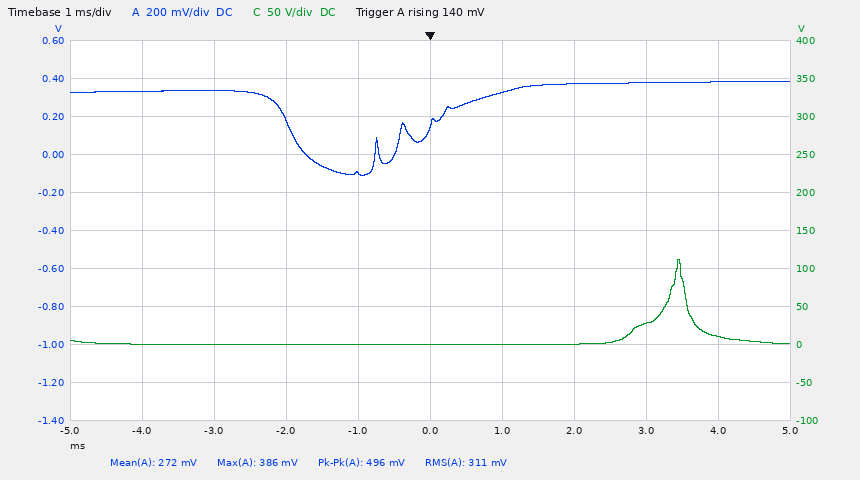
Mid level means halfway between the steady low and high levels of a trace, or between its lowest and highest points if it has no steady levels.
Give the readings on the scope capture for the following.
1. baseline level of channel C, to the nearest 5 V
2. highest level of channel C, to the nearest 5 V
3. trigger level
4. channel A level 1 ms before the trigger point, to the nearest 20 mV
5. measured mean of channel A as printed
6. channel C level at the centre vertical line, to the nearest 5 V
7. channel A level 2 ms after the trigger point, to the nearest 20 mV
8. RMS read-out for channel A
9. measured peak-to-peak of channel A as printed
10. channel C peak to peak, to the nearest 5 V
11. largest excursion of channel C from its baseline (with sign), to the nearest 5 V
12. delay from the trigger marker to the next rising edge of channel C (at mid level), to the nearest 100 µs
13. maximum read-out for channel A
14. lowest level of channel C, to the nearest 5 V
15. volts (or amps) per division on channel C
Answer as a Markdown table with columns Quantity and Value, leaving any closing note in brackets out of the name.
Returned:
| Quantity | Value |
|---|---|
| baseline level of channel C, to the nearest 5 V | 0 V |
| highest level of channel C, to the nearest 5 V | 110 V |
| trigger level | 140 mV |
| channel A level 1 ms before the trigger point, to the nearest 20 mV | -100 mV |
| measured mean of channel A as printed | 272 mV |
| channel C level at the centre vertical line, to the nearest 5 V | 0 V |
| channel A level 2 ms after the trigger point, to the nearest 20 mV | 380 mV |
| RMS read-out for channel A | 311 mV |
| measured peak-to-peak of channel A as printed | 496 mV |
| channel C peak to peak, to the nearest 5 V | 110 V |
| largest excursion of channel C from its baseline (with sign), to the nearest 5 V | +110 V |
| delay from the trigger marker to the next rising edge of channel C (at mid level), to the nearest 100 µs | 3.3 ms |
| maximum read-out for channel A | 386 mV |
| lowest level of channel C, to the nearest 5 V | 0 V |
| volts (or amps) per division on channel C | 50 V |
